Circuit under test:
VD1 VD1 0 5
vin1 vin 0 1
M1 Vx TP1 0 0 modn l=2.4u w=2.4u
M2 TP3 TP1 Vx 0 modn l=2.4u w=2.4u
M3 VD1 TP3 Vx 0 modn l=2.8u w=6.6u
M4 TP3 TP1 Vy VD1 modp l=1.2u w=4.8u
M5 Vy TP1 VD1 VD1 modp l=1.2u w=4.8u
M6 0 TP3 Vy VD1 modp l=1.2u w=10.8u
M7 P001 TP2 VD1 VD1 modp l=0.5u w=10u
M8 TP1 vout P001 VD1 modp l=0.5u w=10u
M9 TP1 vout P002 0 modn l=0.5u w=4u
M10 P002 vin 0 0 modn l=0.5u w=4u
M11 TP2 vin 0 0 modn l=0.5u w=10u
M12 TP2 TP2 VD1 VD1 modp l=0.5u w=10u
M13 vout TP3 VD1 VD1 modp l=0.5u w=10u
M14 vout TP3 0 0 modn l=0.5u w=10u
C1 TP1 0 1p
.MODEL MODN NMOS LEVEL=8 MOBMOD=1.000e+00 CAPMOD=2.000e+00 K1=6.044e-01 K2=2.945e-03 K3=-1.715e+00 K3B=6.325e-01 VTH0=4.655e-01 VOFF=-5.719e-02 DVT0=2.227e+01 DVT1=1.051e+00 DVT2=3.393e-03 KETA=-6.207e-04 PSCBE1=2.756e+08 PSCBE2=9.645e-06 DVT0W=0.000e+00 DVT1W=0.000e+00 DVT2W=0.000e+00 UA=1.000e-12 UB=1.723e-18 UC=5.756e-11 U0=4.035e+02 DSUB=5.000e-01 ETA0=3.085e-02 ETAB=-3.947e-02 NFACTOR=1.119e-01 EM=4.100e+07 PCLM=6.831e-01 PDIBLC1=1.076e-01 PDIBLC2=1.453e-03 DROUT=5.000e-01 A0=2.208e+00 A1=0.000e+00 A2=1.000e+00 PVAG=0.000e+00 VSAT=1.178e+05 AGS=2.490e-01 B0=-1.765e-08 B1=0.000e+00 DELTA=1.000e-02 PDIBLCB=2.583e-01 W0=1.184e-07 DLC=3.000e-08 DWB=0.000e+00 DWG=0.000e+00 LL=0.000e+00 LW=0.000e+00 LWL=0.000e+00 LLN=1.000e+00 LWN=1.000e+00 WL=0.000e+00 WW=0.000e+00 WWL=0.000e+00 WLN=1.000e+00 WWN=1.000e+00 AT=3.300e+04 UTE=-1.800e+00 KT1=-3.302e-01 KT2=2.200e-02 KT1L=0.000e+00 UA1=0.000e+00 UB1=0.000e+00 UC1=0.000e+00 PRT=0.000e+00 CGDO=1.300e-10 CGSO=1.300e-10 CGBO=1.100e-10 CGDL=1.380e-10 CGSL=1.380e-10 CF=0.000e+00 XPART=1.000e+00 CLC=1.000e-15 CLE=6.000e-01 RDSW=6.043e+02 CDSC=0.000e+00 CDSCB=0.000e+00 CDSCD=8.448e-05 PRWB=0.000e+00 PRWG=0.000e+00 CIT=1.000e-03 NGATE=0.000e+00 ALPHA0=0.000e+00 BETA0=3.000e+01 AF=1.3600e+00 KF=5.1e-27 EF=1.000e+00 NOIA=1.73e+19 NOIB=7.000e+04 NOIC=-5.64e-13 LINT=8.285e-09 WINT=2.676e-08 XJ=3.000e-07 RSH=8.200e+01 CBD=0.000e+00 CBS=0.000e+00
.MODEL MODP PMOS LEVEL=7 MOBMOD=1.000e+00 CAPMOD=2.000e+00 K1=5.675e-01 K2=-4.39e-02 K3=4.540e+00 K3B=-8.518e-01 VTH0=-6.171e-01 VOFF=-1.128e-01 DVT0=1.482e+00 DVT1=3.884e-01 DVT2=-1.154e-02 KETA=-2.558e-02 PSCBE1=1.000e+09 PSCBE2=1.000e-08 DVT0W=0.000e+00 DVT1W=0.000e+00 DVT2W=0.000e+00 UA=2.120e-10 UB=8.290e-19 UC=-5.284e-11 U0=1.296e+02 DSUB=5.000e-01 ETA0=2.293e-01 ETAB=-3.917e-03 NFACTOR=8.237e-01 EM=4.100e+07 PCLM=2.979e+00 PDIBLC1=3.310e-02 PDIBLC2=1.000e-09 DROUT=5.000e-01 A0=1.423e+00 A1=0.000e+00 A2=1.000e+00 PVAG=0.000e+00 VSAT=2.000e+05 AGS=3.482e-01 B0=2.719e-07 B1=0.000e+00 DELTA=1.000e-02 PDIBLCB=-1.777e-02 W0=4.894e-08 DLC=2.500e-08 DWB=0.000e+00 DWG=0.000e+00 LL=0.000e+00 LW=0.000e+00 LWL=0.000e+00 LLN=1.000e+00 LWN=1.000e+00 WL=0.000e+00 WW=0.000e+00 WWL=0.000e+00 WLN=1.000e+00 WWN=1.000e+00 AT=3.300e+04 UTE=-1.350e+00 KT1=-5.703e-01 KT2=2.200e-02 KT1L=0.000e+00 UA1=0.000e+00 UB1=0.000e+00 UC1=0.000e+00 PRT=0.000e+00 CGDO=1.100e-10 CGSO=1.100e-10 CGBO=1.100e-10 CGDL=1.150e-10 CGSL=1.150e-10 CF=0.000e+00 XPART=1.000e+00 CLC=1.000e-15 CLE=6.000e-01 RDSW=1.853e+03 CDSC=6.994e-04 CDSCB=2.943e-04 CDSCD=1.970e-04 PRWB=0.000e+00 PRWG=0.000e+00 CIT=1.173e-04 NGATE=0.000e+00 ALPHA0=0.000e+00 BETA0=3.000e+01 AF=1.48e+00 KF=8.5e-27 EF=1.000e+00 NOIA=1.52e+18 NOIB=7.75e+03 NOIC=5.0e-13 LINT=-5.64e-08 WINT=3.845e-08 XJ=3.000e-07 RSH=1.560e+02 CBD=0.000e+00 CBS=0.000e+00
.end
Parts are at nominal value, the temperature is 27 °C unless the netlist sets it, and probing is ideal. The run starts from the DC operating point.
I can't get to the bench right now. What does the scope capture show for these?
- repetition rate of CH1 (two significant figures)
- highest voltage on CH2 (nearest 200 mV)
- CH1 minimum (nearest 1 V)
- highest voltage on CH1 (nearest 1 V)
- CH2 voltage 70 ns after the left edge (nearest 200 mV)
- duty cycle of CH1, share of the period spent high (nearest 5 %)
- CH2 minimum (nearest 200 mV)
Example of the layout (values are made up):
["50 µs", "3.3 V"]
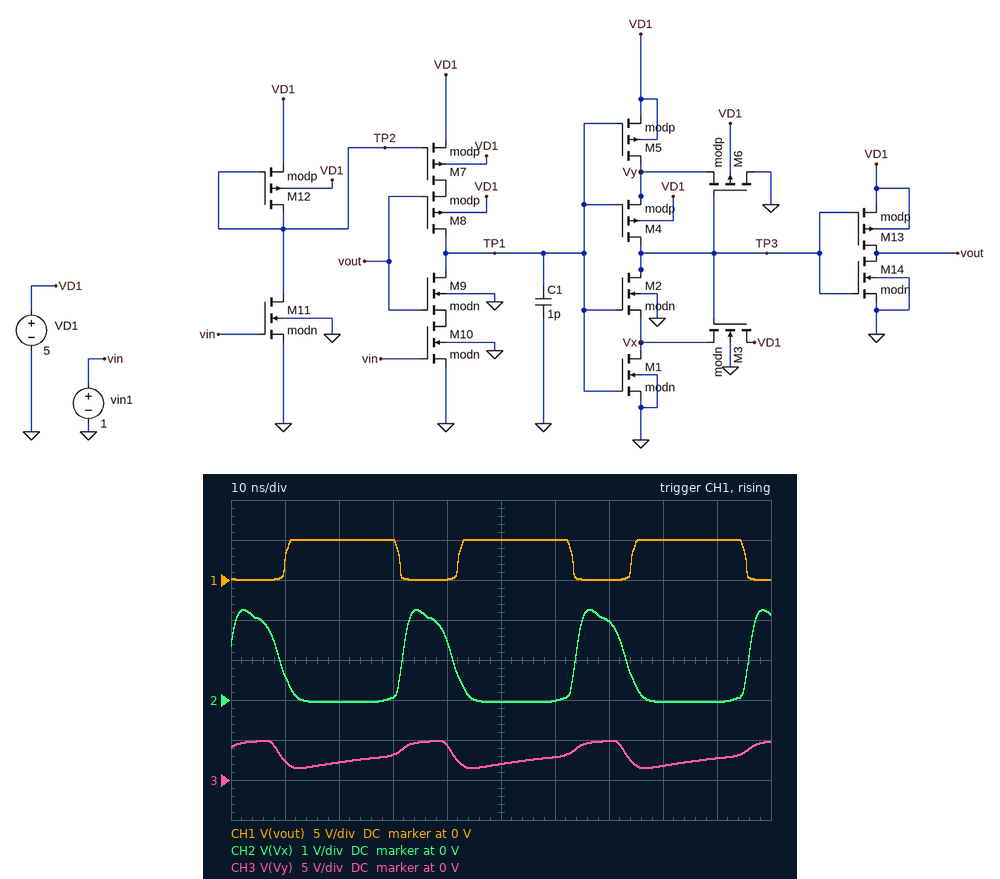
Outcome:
["31 MHz", "2.2 V", "0 V", "5 V", "2.0 V", "65 %", "0 V"]
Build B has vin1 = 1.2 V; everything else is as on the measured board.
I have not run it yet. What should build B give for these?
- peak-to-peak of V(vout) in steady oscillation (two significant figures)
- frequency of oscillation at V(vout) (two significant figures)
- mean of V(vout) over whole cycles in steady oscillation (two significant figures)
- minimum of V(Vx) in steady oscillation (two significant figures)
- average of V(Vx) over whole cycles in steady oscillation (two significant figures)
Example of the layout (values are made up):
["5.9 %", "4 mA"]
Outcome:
["5.0 V", "45 MHz", "3.0 V", "-87 mV", "640 mV"]
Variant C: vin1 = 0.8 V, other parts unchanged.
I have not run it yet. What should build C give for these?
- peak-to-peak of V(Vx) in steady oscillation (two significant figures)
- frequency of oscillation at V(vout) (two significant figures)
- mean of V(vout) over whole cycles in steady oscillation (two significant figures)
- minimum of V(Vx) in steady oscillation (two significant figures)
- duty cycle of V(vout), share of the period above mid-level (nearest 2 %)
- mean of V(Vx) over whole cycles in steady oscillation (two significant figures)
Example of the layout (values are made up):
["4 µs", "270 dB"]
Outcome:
["2.5 V", "16 MHz", "3.7 V", "-27 mV", "76 %", "490 mV"]
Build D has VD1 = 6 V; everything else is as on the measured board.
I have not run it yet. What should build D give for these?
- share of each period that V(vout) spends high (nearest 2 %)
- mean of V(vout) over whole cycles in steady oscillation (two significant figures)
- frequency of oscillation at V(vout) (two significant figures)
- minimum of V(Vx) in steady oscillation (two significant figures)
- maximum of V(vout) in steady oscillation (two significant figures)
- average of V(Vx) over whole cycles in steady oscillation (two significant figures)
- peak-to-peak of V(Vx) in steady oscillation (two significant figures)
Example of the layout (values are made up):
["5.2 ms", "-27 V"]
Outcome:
["70 %", "4.1 V", "32 MHz", "-71 mV", "6.0 V", "610 mV", "2.5 V"]
